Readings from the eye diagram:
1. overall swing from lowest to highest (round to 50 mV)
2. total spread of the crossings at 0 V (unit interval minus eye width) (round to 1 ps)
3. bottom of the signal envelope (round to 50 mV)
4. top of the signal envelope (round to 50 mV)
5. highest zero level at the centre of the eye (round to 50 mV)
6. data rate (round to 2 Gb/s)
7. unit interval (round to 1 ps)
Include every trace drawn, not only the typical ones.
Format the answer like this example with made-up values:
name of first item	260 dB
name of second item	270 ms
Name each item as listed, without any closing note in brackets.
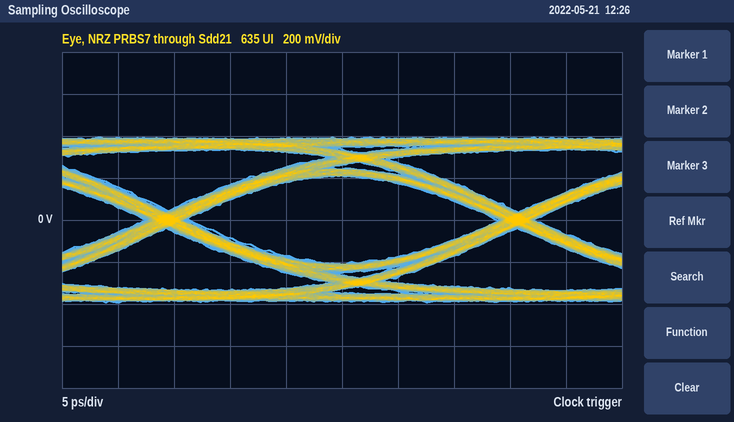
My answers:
overall swing from lowest to highest	800 mV
total spread of the crossings at 0 V (unit interval minus eye width)	4 ps
bottom of the signal envelope	-400 mV
top of the signal envelope	400 mV
highest zero level at the centre of the eye	-200 mV
data rate	32 Gb/s
unit interval	31 ps
